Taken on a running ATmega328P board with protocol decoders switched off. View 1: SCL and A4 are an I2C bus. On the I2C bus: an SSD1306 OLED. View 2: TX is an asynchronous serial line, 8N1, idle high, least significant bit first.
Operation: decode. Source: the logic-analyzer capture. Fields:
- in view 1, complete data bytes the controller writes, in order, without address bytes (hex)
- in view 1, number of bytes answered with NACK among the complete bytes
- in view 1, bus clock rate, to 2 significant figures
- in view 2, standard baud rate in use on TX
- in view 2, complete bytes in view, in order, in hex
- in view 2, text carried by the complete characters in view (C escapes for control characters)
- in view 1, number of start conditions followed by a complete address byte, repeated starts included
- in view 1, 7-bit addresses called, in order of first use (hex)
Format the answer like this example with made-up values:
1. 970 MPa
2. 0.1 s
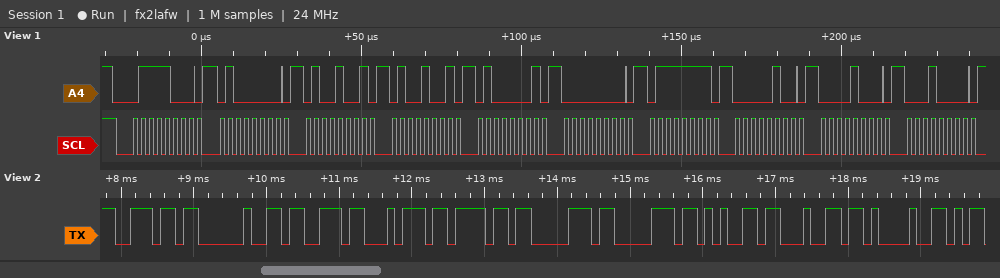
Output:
1. 40 49 49 41 00 7F 04 08 10
2. 0
3. 400 kHz
4. 9600 baud
5. 6E 20 73 74 6F 70 70 65 64 21
6. "n stopped!"
7. 1
8. 0x3C
